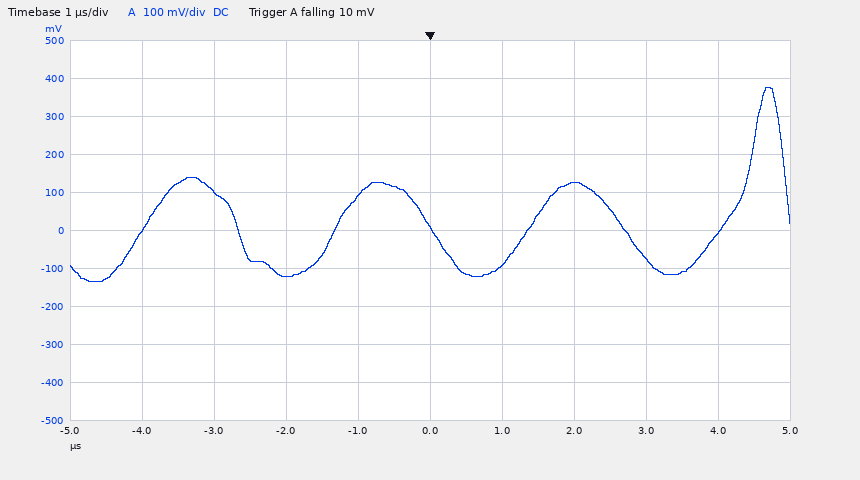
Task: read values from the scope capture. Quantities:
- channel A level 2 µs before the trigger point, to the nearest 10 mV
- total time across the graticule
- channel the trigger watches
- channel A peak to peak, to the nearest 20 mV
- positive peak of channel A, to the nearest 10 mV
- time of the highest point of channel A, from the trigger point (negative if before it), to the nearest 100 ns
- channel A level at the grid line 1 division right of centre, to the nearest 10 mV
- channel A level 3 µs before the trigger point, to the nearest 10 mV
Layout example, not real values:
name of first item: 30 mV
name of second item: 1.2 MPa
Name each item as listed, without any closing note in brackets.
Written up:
channel A level 2 µs before the trigger point, to the nearest 10 mV: -120 mV
total time across the graticule: 10 µs
channel the trigger watches: channel A
channel A peak to peak, to the nearest 20 mV: 520 mV
positive peak of channel A, to the nearest 10 mV: 380 mV
time of the highest point of channel A, from the trigger point (negative if before it), to the nearest 100 ns: +4.7 µs
channel A level at the grid line 1 division right of centre, to the nearest 10 mV: -90 mV
channel A level 3 µs before the trigger point, to the nearest 10 mV: 100 mV
